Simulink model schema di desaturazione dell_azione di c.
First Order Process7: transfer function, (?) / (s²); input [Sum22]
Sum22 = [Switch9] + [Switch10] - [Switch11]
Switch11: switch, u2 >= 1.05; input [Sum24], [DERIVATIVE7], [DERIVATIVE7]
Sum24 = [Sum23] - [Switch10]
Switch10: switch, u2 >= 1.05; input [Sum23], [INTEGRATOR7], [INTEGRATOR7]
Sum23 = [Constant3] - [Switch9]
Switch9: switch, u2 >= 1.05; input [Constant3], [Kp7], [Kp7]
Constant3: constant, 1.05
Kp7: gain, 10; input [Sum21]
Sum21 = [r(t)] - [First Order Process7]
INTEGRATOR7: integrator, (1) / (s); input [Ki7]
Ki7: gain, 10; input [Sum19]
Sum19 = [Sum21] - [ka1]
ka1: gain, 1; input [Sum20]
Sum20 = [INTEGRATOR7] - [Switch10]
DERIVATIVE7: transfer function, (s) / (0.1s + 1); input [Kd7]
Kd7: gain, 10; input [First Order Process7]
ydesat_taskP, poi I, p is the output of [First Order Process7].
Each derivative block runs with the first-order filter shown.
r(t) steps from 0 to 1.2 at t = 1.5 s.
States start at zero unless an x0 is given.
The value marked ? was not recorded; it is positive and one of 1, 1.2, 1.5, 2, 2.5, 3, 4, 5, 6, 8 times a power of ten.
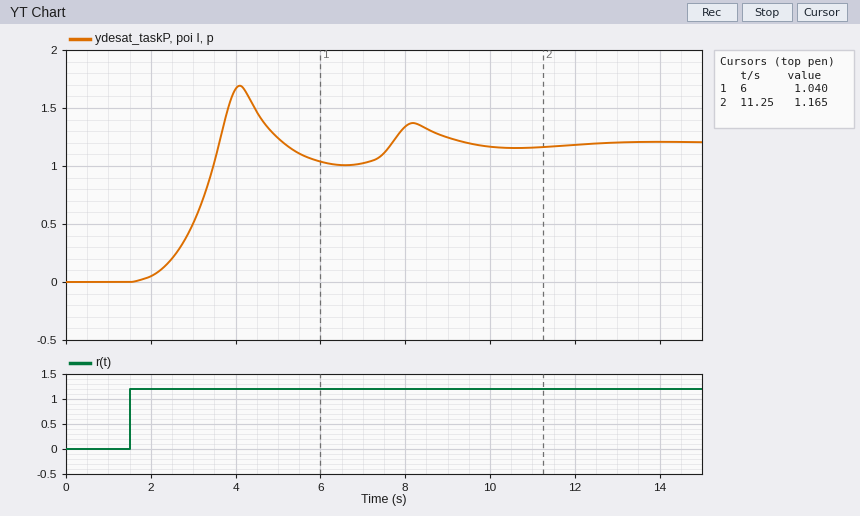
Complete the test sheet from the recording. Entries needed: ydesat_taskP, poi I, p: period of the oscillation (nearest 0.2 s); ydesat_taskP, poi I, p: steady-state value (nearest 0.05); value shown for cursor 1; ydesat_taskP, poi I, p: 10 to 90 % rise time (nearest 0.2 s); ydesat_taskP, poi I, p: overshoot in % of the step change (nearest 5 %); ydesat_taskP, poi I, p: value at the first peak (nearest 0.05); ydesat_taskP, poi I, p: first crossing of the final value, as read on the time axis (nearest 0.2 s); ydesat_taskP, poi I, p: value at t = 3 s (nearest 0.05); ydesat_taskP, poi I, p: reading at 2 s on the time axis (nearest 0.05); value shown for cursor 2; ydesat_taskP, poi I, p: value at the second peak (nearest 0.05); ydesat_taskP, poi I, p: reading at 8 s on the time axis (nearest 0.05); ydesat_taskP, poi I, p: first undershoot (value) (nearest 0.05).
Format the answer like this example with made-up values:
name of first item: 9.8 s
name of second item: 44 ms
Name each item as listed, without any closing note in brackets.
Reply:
ydesat_taskP, poi I, p: period of the oscillation: 4.0 s
ydesat_taskP, poi I, p: steady-state value: 1.20
value shown for cursor 1: 1.040
ydesat_taskP, poi I, p: 10 to 90 % rise time: 1.2 s
ydesat_taskP, poi I, p: overshoot in % of the step change: 40 %
ydesat_taskP, poi I, p: value at the first peak: 1.70
ydesat_taskP, poi I, p: first crossing of the final value, as read on the time axis: 3.6 s
ydesat_taskP, poi I, p: value at t = 3 s: 0.50
ydesat_taskP, poi I, p: reading at 2 s on the time axis: 0.05
value shown for cursor 2: 1.165
ydesat_taskP, poi I, p: value at the second peak: 1.35
ydesat_taskP, poi I, p: reading at 8 s on the time axis: 1.35
ydesat_taskP, poi I, p: first undershoot (value): 1.00
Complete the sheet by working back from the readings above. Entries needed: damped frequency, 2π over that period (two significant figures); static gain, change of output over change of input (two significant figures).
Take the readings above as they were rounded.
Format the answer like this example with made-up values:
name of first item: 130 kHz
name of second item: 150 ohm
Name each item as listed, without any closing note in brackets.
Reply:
damped frequency, 2π over that period: 1.6 rad/s
static gain, change of output over change of input: 1.0
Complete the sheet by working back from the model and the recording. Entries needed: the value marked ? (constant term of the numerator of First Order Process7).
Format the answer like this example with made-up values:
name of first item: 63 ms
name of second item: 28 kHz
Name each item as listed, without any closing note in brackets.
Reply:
the value marked ?: 0.5
